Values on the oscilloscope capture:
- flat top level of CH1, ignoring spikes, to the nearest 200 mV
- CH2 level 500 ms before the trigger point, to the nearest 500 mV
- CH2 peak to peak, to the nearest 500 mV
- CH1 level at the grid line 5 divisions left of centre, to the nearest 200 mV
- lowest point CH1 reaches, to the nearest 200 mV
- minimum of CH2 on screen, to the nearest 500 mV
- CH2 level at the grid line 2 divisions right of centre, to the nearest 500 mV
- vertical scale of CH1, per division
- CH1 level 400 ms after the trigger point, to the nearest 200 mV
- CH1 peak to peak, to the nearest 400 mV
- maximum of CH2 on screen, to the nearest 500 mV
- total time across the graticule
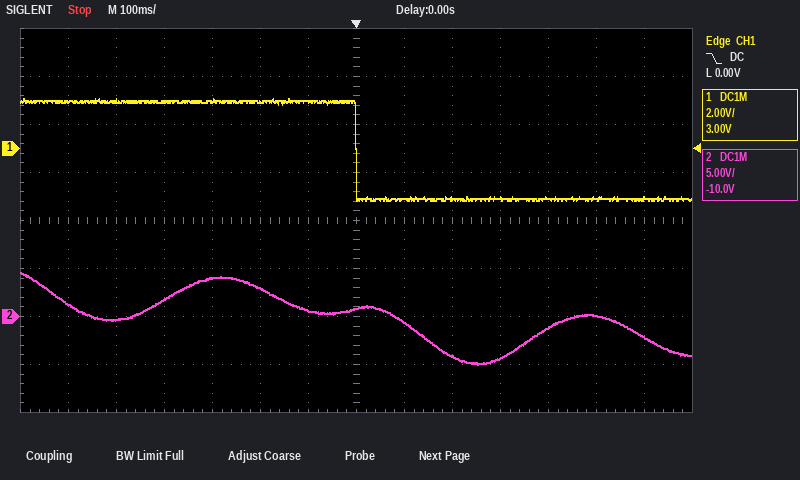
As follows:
2.0 V
-500 mV
9.5 V
2.0 V
-2.2 V
-5.0 V
-4.0 V
2 V
-2.0 V
4.4 V
4.5 V
1.4 s
